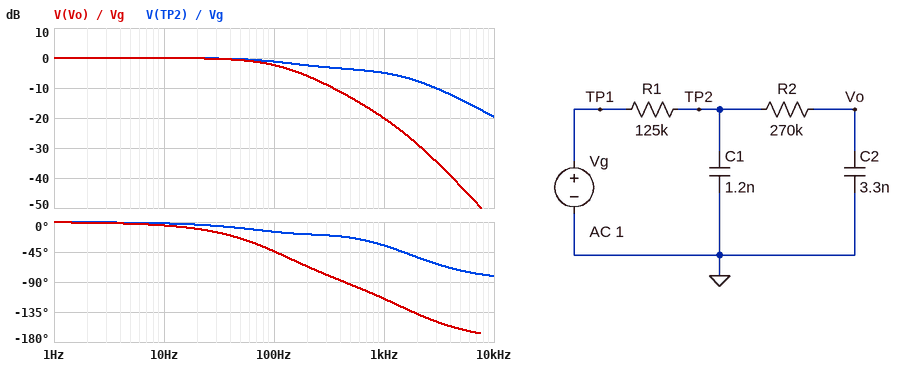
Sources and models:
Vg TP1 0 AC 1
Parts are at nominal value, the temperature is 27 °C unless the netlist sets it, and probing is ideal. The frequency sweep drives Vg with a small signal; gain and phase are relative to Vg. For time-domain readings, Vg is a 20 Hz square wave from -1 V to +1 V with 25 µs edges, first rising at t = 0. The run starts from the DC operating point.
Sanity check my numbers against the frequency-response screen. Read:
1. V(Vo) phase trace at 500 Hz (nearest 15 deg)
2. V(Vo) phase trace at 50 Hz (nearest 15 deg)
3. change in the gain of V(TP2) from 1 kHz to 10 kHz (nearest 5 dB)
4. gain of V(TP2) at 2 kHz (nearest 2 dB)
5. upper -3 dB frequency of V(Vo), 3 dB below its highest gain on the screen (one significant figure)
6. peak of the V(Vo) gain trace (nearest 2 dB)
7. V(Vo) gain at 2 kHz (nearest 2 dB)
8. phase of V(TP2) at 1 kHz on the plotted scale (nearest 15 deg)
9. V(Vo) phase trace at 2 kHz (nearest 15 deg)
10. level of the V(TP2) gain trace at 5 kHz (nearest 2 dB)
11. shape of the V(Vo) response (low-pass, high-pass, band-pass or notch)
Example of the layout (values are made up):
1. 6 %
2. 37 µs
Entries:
1. -90 deg
2. -30 deg
3. -15 dB
4. -8 dB
5. 100 Hz
6. 0 dB
7. -28 dB
8. -30 deg
9. -135 deg
10. -14 dB
11. low-pass
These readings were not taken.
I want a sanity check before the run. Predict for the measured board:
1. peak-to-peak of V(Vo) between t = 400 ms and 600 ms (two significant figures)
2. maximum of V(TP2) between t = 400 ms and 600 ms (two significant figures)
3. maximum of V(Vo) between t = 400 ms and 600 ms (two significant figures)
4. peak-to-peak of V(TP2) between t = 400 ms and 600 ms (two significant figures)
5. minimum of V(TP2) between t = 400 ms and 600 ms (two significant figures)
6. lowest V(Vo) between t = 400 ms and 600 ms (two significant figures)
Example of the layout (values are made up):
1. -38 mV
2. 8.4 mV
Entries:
1. 2.0 V
2. 1.0 V
3. 1.0 V
4. 2.0 V
5. -1.0 V
6. -1.0 V
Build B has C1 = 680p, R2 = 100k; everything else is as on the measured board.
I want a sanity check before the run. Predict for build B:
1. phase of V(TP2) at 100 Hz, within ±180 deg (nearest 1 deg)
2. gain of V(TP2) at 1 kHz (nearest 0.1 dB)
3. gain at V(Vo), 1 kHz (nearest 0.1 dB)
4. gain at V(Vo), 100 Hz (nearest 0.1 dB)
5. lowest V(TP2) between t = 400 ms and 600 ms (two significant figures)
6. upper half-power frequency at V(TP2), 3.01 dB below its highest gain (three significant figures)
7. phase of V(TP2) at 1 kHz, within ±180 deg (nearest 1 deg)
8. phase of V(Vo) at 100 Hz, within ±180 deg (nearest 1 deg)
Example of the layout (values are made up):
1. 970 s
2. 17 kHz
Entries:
1. -16 deg
2. -7.1 dB
3. -14.3 dB
4. -1.0 dB
5. -1.0 V
6. 248 Hz
7. -27 deg
8. -28 deg
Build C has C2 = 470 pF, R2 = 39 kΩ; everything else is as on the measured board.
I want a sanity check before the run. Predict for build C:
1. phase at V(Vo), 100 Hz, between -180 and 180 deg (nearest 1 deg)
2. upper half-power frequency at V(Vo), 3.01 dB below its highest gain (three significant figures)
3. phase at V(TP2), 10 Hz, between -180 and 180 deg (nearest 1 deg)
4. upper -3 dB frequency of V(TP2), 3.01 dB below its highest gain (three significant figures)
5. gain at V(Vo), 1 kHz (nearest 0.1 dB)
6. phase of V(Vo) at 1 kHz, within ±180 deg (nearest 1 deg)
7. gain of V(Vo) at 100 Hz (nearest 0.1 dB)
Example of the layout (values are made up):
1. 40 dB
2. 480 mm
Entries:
1. -8 deg
2. 740 Hz
3. -1 deg
4. 746 Hz
5. -4.5 dB
6. -58 deg
7. -0.1 dB
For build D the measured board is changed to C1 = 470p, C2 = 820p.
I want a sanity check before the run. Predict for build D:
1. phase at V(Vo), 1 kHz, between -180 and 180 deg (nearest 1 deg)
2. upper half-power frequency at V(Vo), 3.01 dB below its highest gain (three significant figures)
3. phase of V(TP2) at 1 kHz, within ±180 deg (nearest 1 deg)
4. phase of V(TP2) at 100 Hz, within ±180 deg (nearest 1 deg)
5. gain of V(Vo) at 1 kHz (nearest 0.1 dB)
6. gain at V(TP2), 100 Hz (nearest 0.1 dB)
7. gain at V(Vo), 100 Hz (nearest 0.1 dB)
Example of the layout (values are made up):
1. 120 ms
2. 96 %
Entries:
1. -79 deg
2. 456 Hz
3. -24 deg
4. -6 deg
5. -7.8 dB
6. -0.1 dB
7. -0.2 dB
